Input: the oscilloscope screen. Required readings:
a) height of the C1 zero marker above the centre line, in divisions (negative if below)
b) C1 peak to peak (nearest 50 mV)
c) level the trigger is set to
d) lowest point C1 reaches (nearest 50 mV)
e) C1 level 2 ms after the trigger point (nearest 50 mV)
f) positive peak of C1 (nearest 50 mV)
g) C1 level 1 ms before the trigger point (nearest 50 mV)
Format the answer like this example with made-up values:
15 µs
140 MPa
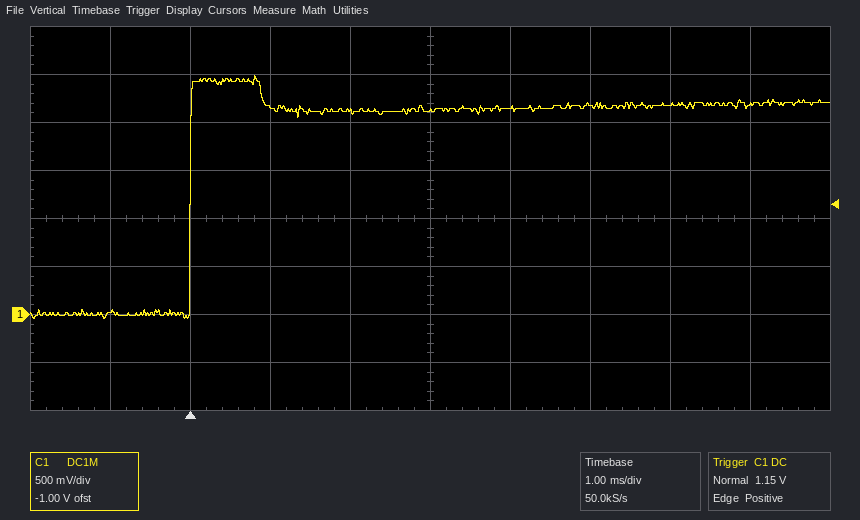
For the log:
-2.0 div
2.55 V
1.15 V
-50 mV
2.10 V
2.50 V
0 mV
